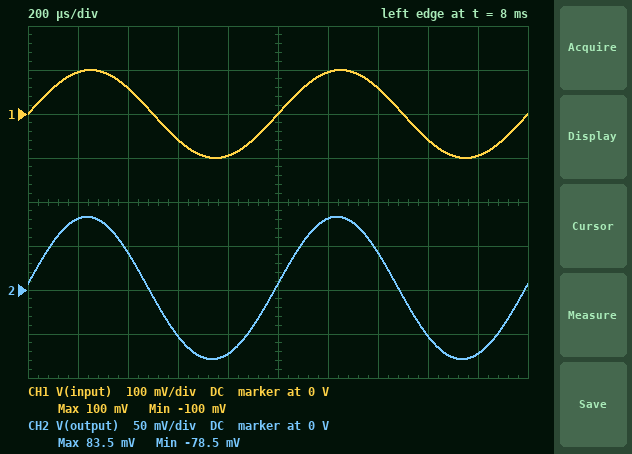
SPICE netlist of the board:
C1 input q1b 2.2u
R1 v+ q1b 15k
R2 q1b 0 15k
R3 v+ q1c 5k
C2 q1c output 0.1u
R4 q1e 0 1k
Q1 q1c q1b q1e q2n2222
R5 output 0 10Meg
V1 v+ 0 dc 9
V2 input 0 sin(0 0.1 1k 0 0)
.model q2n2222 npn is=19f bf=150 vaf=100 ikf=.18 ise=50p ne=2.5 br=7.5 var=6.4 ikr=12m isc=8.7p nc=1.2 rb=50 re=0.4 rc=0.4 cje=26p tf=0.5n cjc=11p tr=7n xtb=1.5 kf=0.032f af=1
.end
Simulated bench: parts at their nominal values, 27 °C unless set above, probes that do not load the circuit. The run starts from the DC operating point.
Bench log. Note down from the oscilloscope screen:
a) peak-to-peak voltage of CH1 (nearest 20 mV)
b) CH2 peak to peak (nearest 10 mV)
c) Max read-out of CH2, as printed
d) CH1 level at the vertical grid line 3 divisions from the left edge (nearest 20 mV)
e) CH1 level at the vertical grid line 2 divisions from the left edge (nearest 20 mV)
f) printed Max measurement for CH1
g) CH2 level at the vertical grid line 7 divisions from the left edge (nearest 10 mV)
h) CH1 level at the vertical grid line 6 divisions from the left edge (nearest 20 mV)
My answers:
200 mV
160 mV
83.5 mV
-60 mV
60 mV
100 mV
40 mV
100 mV
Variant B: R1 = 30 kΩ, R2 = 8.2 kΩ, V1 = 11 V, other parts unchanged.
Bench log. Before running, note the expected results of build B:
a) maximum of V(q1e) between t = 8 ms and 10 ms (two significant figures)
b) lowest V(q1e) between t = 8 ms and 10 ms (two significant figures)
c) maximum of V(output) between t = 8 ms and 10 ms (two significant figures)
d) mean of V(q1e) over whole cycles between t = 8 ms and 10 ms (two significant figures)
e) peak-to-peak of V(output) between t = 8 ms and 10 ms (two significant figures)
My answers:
1.7 V
1.5 V
490 mV
1.6 V
970 mV
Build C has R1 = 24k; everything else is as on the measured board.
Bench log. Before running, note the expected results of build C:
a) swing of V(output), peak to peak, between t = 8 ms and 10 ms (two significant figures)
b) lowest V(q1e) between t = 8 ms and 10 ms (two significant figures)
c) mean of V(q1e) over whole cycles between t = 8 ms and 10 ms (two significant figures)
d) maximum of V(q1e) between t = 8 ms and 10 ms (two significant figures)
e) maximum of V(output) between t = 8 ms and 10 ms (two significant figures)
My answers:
110 mV
1.5 V
1.6 V
1.7 V
73 mV
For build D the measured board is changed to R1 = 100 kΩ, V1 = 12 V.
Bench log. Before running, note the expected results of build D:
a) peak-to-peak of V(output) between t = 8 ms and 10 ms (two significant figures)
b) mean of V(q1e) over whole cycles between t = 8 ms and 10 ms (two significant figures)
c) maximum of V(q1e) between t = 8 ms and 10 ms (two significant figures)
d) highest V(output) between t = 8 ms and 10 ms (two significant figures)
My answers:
960 mV
840 mV
940 mV
480 mV
